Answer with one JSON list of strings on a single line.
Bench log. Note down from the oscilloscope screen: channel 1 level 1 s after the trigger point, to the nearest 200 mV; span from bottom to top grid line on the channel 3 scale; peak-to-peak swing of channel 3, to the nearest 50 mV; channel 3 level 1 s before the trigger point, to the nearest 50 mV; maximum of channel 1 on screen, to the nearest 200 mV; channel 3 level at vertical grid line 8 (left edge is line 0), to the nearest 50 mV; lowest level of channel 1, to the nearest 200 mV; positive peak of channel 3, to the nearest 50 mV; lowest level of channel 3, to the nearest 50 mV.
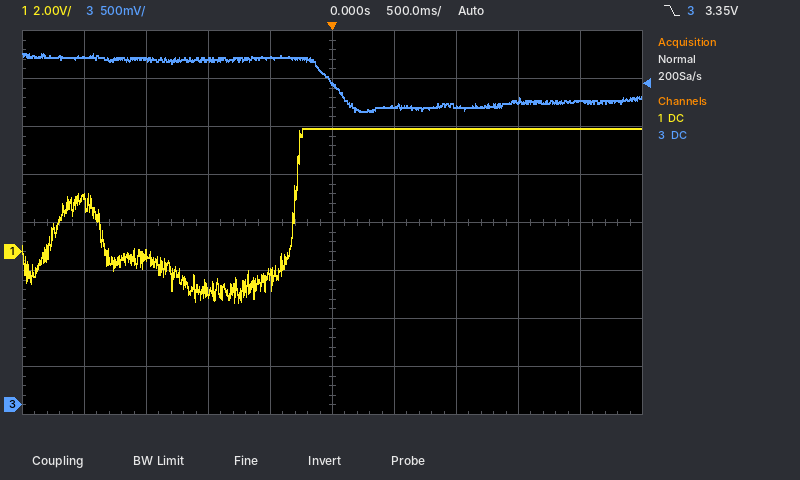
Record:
["5.2 V", "4 V", "600 mV", "3.60 V", "5.2 V", "3.15 V", "-2.2 V", "3.65 V", "3.05 V"]
